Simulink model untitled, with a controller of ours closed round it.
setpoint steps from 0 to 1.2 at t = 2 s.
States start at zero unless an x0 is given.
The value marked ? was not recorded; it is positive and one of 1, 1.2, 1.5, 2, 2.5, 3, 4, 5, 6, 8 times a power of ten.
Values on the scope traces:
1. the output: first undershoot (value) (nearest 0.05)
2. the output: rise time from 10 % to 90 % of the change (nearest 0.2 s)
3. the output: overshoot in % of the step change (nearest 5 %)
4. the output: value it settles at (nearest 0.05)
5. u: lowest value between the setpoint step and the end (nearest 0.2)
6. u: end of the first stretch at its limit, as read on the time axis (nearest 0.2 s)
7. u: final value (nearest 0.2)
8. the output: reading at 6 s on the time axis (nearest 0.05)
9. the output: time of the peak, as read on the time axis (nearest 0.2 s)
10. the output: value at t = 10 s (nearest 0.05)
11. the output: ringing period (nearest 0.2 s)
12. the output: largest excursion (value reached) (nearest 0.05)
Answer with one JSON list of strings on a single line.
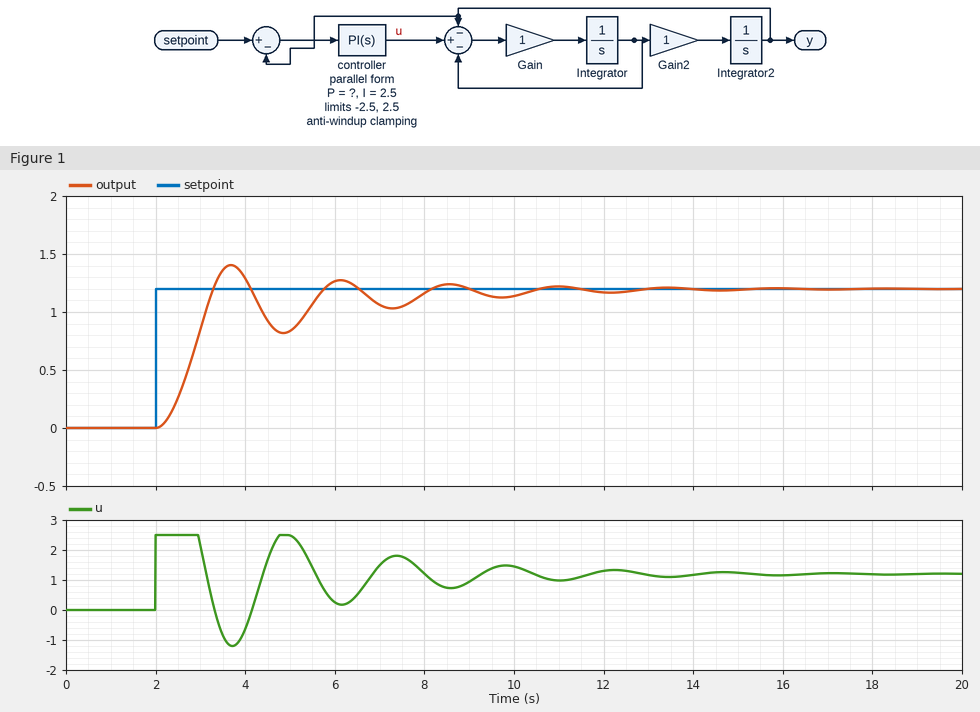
["0.80", "0.8 s", "15 %", "1.20", "-1.2", "3.0 s", "1.2", "1.25", "3.6 s", "1.15", "2.4 s", "1.40"]
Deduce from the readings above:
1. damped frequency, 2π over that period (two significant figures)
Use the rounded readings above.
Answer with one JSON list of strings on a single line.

["2.6 rad/s"]
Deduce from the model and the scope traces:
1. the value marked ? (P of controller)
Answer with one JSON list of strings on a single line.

["6"]
